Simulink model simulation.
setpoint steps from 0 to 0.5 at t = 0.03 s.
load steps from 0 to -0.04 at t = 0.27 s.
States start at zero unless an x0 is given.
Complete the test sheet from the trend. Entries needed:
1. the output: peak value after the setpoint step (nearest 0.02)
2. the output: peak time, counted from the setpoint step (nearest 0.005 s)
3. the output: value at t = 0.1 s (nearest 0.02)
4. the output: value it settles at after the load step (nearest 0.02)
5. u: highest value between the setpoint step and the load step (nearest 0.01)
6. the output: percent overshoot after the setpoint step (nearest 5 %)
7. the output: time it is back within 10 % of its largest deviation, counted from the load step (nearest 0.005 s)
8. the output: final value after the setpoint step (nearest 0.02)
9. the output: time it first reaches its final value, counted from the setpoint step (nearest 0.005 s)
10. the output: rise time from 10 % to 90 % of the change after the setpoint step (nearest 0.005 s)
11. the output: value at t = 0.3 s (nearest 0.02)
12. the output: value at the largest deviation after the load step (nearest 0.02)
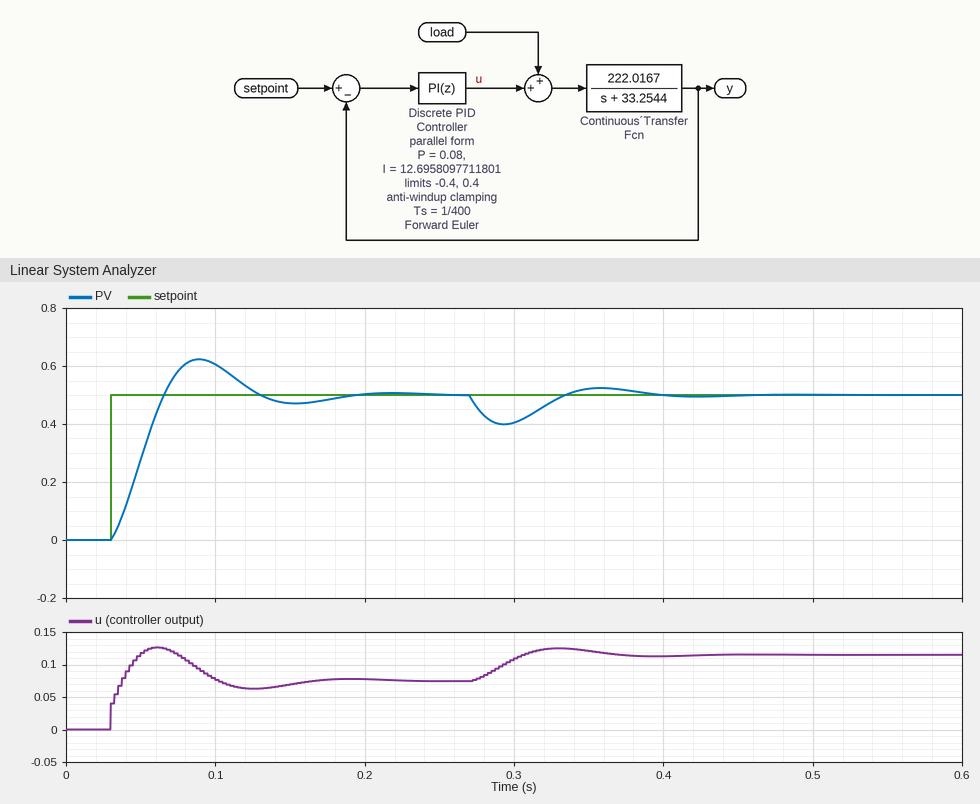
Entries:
0.62
0.060 s
0.60
0.50
0.13
25 %
0.115 s
0.50
0.035 s
0.025 s
0.40
0.40
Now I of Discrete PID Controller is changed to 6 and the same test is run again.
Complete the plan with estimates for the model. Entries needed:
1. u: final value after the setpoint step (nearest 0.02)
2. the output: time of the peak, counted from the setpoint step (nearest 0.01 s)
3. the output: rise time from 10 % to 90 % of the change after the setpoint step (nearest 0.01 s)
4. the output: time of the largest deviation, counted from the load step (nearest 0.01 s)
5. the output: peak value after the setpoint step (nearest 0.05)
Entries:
0.08
0.10 s
0.05 s
0.03 s
0.55
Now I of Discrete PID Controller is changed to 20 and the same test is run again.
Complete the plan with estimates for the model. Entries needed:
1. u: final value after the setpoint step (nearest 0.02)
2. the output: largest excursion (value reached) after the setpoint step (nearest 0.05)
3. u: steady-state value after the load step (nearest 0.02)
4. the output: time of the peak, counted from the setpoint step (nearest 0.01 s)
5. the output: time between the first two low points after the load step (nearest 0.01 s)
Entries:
0.08
0.70
0.12
0.05 s
0.10 s
